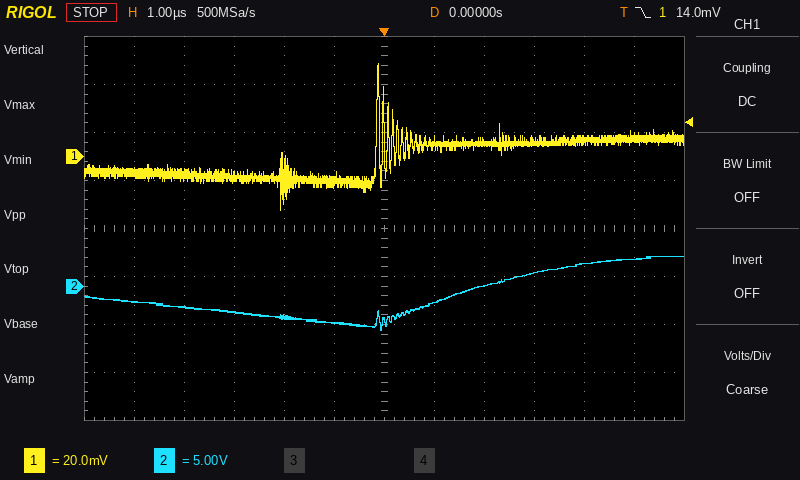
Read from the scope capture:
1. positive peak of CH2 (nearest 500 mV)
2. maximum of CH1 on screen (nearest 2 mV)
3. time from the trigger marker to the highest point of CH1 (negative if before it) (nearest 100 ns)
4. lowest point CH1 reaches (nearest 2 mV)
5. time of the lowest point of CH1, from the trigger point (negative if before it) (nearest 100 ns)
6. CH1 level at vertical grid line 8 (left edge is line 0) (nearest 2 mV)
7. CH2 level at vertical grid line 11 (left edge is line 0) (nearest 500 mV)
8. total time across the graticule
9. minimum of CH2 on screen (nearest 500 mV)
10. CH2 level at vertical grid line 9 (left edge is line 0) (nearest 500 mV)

3.0 V
38 mV
-100 ns
-22 mV
-2.1 µs
6 mV
3.0 V
12 µs
-4.5 V
1.5 V
